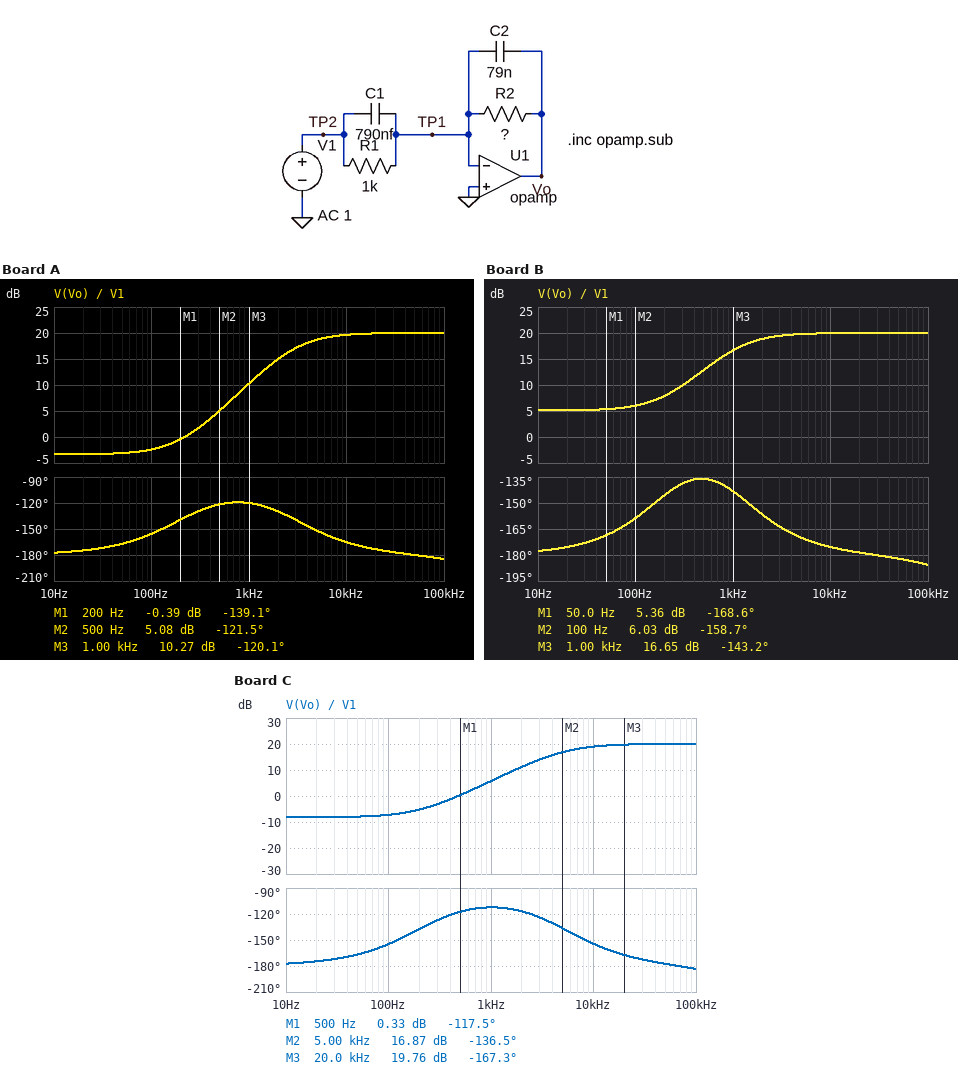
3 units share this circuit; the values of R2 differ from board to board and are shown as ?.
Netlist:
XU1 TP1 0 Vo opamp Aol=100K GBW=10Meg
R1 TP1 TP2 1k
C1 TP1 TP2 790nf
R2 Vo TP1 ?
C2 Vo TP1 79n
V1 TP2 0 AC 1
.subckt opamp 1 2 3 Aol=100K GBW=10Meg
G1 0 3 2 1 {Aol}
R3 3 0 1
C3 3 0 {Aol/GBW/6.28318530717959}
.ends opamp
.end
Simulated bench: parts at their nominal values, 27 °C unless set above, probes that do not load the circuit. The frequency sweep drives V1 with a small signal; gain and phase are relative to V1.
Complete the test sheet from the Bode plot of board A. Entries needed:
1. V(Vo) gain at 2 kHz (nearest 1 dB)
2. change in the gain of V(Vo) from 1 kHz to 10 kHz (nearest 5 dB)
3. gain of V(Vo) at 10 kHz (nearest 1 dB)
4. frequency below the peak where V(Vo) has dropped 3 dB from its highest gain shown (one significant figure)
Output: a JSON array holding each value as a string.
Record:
["15 dB", "10 dB", "20 dB", "3 kHz"]
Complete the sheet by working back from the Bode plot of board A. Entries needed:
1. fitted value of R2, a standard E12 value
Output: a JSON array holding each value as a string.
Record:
["680 Ω"]
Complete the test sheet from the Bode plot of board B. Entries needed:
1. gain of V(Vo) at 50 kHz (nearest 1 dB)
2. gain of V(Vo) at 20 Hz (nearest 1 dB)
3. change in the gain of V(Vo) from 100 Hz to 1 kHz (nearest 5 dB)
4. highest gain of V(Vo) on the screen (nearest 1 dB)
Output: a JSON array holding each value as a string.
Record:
["20 dB", "5 dB", "10 dB", "20 dB"]
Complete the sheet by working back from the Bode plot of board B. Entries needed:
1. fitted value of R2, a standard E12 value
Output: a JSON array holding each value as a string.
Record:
["1.8 kΩ"]
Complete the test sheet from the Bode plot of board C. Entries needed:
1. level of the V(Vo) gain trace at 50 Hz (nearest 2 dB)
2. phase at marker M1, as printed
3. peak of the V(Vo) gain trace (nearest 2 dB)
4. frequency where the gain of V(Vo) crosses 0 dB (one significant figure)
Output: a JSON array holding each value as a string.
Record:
["-8 dB", "-117.5 deg", "20 dB", "500 Hz"]
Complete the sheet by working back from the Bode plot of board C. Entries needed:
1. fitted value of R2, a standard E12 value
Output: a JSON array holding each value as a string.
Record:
["390 Ω"]
